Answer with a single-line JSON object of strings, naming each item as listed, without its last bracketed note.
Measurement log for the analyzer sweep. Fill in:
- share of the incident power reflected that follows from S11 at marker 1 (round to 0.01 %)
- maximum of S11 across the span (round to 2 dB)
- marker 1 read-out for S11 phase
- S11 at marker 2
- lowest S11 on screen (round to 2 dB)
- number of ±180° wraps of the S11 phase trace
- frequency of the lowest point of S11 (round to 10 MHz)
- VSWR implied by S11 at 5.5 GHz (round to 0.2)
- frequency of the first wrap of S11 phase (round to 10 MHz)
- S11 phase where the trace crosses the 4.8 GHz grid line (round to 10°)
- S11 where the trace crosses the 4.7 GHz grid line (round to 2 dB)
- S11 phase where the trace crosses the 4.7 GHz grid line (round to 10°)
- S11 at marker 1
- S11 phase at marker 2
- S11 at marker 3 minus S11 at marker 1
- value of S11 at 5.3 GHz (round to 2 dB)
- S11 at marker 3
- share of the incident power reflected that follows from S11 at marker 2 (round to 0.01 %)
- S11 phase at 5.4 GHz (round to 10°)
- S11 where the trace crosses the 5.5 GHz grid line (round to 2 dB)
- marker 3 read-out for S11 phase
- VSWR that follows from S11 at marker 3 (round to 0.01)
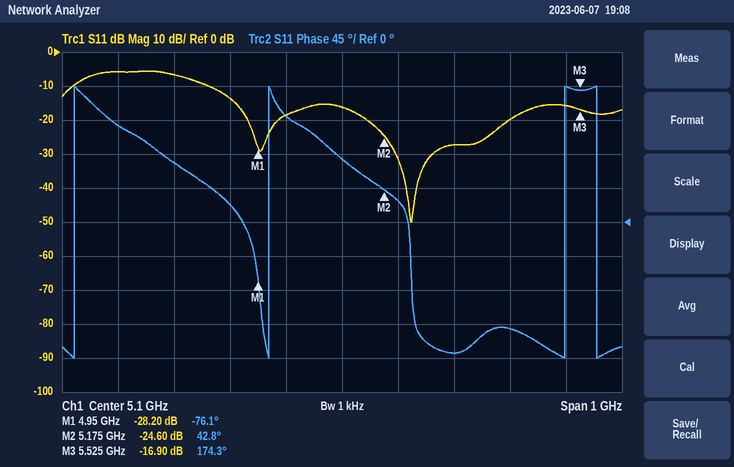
{"share of the incident power reflected that follows from S11 at marker 1": "0.15 %", "maximum of S11 across the span": "-6 dB", "marker 1 read-out for S11 phase": "-76.1°", "S11 at marker 2": "-24.60 dB", "lowest S11 on screen": "-50 dB", "number of ±180° wraps of the S11 phase trace": "4", "frequency of the lowest point of S11": "5.22 GHz", "VSWR implied by S11 at 5.5 GHz": "1.4", "frequency of the first wrap of S11 phase": "4.62 GHz", "S11 phase where the trace crosses the 4.8 GHz grid line": "80°", "S11 where the trace crosses the 4.7 GHz grid line": "-6 dB", "S11 phase where the trace crosses the 4.7 GHz grid line": "130°", "S11 at marker 1": "-28.20 dB", "S11 phase at marker 2": "42.8°", "S11 at marker 3 minus S11 at marker 1": "11.30 dB", "value of S11 at 5.3 GHz": "-28 dB", "S11 at marker 3": "-16.90 dB", "share of the incident power reflected that follows from S11 at marker 2": "0.35 %", "S11 phase at 5.4 GHz": "-140°", "S11 where the trace crosses the 5.5 GHz grid line": "-16 dB", "marker 3 read-out for S11 phase": "174.3°", "VSWR that follows from S11 at marker 3": "1.33"}
